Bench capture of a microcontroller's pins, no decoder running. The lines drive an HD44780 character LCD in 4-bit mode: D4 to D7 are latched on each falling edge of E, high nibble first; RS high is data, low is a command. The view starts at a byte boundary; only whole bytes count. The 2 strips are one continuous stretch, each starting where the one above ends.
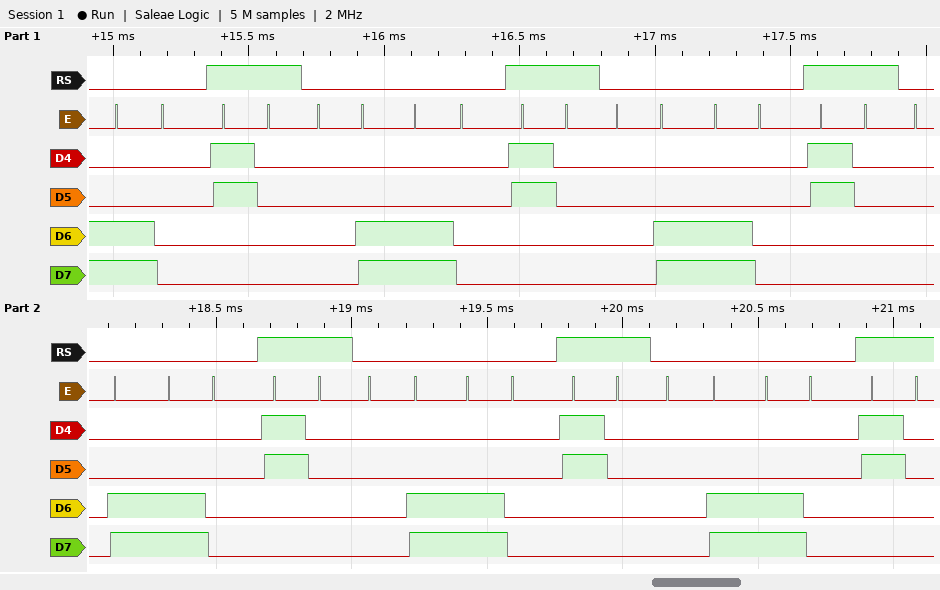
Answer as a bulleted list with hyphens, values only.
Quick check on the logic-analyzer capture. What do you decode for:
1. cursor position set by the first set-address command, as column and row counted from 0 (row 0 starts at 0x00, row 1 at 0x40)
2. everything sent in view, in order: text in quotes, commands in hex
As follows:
- column 0, row 1
- 0xC0 "0" 0x0C 0xC0 "0" 0x0C 0xC0 "0" 0x0C 0xC0 "0" 0x0C 0xC0 "0" 0x0C 0xC0 "0"
